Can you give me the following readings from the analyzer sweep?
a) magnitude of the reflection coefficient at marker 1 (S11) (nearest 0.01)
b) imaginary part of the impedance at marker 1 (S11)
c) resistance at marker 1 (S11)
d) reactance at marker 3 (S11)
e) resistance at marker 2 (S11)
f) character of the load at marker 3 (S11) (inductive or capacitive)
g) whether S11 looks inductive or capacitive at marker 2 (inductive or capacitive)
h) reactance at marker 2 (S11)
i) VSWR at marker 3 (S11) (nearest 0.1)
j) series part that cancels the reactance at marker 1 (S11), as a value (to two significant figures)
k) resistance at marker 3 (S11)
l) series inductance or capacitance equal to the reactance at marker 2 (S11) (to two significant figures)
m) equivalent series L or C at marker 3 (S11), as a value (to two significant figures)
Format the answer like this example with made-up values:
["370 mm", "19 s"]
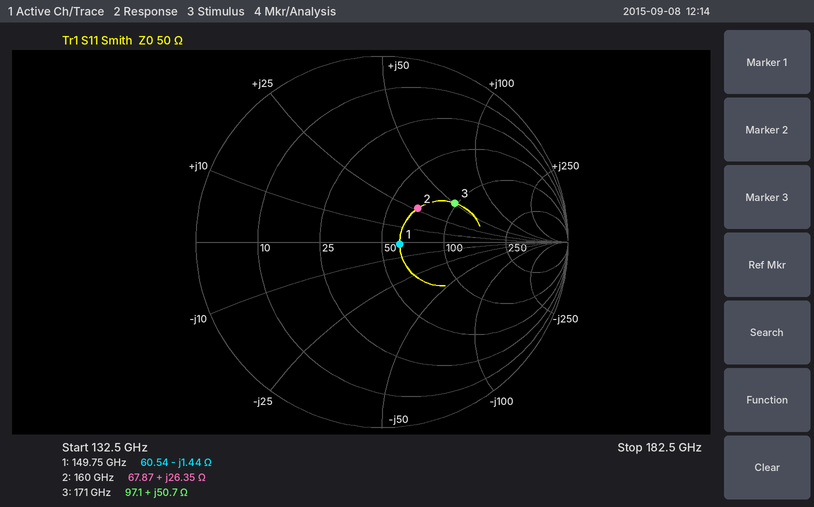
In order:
["0.10", "-1.44 Ω", "60.54 Ω", "+50.7 Ω", "67.87 Ω", "inductive", "inductive", "+26.35 Ω", "2.6", "1.5 pH", "97.1 Ω", "26 pH", "47 pH"]
